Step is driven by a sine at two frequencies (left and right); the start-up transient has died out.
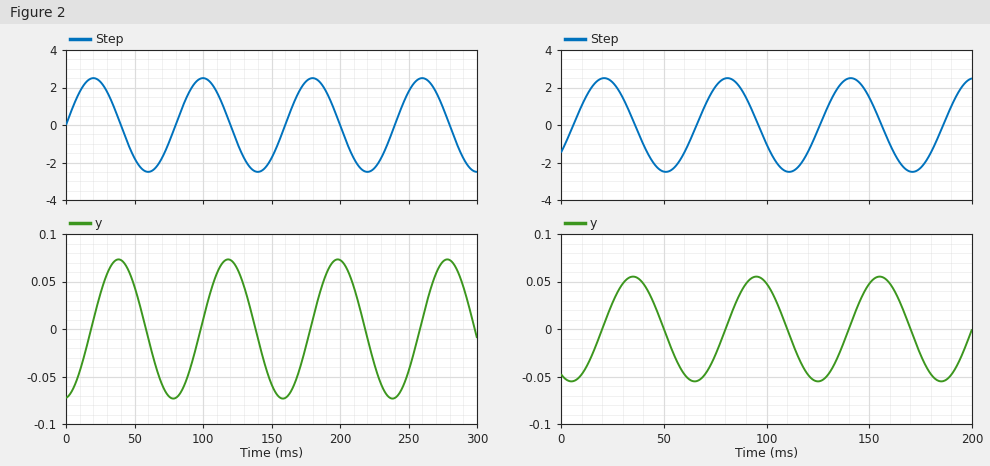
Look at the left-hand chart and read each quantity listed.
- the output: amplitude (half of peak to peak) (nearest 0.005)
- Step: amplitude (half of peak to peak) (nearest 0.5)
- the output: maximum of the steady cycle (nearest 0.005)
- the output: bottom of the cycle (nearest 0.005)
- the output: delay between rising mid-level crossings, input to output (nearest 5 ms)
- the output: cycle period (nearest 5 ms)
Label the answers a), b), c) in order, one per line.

a) 0.075
b) 2.5
c) 0.075
d) -0.075
e) 20 ms
f) 80 ms
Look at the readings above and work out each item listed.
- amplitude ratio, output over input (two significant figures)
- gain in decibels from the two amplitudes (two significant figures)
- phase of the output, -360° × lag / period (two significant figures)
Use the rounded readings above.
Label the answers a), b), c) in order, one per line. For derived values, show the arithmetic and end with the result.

a) 0.075 / 2.5 = 0.030
b) 20 log10(0.075 / 2.5) = -30 dB
c) -360 × 20 / 80 = -90°
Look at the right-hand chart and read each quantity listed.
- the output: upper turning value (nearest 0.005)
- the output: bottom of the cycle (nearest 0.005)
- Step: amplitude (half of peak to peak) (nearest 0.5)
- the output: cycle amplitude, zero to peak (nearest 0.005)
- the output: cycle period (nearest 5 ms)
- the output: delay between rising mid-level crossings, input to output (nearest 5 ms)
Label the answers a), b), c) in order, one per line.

a) 0.055
b) -0.055
c) 2.5
d) 0.055
e) 60 ms
f) 15 ms
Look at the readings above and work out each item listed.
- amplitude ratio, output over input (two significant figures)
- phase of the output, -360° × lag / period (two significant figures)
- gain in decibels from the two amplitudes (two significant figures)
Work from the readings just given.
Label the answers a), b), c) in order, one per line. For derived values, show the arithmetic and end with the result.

a) 0.055 / 2.5 = 0.022
b) -360 × 15 / 60 = -90°
c) 20 log10(0.055 / 2.5) = -33 dB
